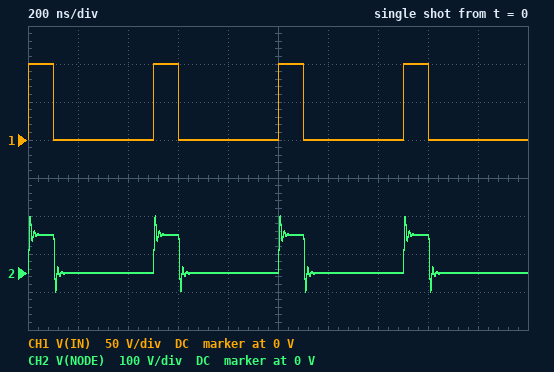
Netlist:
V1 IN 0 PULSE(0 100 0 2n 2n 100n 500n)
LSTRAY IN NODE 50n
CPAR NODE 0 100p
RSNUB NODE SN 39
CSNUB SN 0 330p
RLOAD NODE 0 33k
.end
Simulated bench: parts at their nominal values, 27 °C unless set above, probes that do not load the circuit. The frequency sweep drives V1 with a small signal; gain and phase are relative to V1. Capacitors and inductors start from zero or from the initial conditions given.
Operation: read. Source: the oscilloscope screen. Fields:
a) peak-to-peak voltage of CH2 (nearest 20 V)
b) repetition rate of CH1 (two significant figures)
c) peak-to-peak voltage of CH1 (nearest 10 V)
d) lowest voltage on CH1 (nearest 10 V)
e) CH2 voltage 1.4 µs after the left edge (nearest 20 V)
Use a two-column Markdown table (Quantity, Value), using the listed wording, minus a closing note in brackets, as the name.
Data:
| Quantity | Value |
|---|---|
| peak-to-peak voltage of CH2 | 200 V |
| repetition rate of CH1 | 2.0 MHz |
| peak-to-peak voltage of CH1 | 100 V |
| lowest voltage on CH1 | 0 V |
| CH2 voltage 1.4 µs after the left edge | 0 V |
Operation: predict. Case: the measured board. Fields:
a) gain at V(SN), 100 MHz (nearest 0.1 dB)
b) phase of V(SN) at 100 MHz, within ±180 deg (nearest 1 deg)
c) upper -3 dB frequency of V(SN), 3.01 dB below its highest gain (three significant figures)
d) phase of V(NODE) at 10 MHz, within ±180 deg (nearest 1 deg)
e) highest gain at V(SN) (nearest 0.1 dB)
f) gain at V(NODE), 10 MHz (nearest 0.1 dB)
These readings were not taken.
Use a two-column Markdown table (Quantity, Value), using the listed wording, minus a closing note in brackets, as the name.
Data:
| Quantity | Value |
|---|---|
| gain at V(SN), 100 MHz | -20.7 dB |
| phase of V(SN) at 100 MHz, within ±180 deg | 134 deg |
| upper -3 dB frequency of V(SN), 3.01 dB below its highest gain | 15.0 MHz |
| phase of V(NODE) at 10 MHz, within ±180 deg | -2 deg |
| highest gain at V(SN) | 0 dB |
| gain at V(NODE), 10 MHz | 0.5 dB |
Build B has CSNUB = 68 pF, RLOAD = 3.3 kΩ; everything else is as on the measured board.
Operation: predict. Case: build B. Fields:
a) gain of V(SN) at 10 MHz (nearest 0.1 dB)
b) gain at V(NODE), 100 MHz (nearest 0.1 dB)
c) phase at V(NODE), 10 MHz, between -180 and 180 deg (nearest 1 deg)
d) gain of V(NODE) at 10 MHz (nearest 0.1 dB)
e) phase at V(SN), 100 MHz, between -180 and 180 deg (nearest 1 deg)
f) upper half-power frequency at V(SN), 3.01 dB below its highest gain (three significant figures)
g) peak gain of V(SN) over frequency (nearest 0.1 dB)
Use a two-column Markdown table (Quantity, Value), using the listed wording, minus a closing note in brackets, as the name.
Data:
| Quantity | Value |
|---|---|
| gain of V(SN) at 10 MHz | 0.2 dB |
| gain at V(NODE), 100 MHz | -3.3 dB |
| phase at V(NODE), 10 MHz, between -180 and 180 deg | 0 deg |
| gain of V(NODE) at 10 MHz | 0.3 dB |
| phase at V(SN), 100 MHz, between -180 and 180 deg | 145 deg |
| upper half-power frequency at V(SN), 3.01 dB below its highest gain | 66.5 MHz |
| peak gain of V(SN) over frequency | 9.1 dB |
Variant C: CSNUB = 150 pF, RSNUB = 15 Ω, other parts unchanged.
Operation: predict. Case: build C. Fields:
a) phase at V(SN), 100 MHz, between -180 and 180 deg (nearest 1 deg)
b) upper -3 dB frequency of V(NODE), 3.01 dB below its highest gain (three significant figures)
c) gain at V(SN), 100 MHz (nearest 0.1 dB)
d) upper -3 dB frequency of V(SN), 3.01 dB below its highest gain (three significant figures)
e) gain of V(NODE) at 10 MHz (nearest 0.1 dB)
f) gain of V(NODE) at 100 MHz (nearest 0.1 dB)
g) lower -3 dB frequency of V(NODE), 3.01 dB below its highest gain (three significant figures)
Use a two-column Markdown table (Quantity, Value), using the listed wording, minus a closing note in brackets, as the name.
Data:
| Quantity | Value |
|---|---|
| phase at V(SN), 100 MHz, between -180 and 180 deg | 161 deg |
| upper -3 dB frequency of V(NODE), 3.01 dB below its highest gain | 54.7 MHz |
| gain at V(SN), 100 MHz | -12.4 dB |
| upper -3 dB frequency of V(SN), 3.01 dB below its highest gain | 53.8 MHz |
| gain of V(NODE) at 10 MHz | 0.4 dB |
| gain of V(NODE) at 100 MHz | -7.6 dB |
| lower -3 dB frequency of V(NODE), 3.01 dB below its highest gain | 36.6 MHz |
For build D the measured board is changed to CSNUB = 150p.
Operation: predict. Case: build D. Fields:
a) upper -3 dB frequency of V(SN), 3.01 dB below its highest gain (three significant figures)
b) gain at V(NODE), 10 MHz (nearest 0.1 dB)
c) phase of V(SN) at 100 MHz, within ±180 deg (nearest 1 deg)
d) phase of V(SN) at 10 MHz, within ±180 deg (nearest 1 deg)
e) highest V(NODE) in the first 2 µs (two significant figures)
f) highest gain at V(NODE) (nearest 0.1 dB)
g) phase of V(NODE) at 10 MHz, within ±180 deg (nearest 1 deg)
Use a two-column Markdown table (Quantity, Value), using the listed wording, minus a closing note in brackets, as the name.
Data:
| Quantity | Value |
|---|---|
| upper -3 dB frequency of V(SN), 3.01 dB below its highest gain | 68.7 MHz |
| gain at V(NODE), 10 MHz | 0.4 dB |
| phase of V(SN) at 100 MHz, within ±180 deg | 138 deg |
| phase of V(SN) at 10 MHz, within ±180 deg | -21 deg |
| highest V(NODE) in the first 2 µs | 160 V |
| highest gain at V(NODE) | 7.7 dB |
| phase of V(NODE) at 10 MHz, within ±180 deg | -1 deg |
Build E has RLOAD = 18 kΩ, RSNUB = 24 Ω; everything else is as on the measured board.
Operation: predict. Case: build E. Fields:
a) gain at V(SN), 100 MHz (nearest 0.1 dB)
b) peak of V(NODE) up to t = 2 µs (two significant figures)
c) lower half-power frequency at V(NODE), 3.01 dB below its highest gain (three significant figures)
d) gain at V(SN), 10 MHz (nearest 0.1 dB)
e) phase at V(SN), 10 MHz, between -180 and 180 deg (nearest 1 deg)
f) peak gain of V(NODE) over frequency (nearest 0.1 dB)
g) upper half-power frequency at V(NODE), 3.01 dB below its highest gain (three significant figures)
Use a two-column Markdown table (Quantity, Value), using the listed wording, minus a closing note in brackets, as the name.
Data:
| Quantity | Value |
|---|---|
| gain at V(SN), 100 MHz | -19.0 dB |
| peak of V(NODE) up to t = 2 µs | 140 V |
| lower half-power frequency at V(NODE), 3.01 dB below its highest gain | 13.8 MHz |
| gain at V(SN), 10 MHz | -0.3 dB |
| phase at V(SN), 10 MHz, between -180 and 180 deg | -28 deg |
| peak gain of V(NODE) over frequency | 4.1 dB |
| upper half-power frequency at V(NODE), 3.01 dB below its highest gain | 70.3 MHz |
